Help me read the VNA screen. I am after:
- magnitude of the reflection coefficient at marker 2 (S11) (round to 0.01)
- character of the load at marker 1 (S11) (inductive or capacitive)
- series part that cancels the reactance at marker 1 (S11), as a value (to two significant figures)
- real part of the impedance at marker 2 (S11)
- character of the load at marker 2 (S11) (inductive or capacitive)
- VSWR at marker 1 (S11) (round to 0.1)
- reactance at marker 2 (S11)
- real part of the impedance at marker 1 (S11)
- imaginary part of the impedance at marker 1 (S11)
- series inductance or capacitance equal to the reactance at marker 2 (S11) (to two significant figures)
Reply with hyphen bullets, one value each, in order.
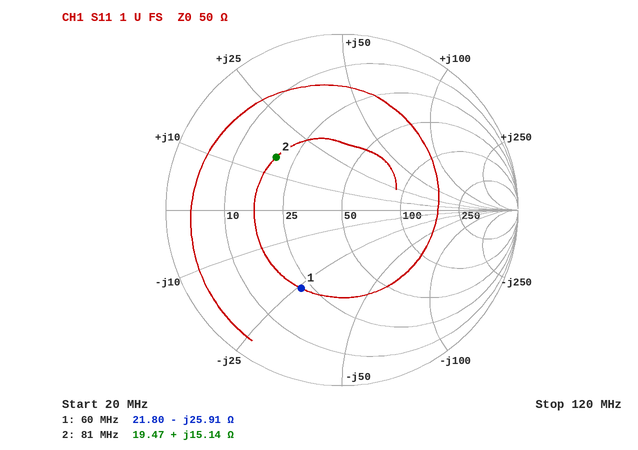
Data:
- 0.48
- capacitive
- 69 nH
- 19.47 Ω
- inductive
- 3.0
- +15.14 Ω
- 21.80 Ω
- -25.91 Ω
- 30 nH
